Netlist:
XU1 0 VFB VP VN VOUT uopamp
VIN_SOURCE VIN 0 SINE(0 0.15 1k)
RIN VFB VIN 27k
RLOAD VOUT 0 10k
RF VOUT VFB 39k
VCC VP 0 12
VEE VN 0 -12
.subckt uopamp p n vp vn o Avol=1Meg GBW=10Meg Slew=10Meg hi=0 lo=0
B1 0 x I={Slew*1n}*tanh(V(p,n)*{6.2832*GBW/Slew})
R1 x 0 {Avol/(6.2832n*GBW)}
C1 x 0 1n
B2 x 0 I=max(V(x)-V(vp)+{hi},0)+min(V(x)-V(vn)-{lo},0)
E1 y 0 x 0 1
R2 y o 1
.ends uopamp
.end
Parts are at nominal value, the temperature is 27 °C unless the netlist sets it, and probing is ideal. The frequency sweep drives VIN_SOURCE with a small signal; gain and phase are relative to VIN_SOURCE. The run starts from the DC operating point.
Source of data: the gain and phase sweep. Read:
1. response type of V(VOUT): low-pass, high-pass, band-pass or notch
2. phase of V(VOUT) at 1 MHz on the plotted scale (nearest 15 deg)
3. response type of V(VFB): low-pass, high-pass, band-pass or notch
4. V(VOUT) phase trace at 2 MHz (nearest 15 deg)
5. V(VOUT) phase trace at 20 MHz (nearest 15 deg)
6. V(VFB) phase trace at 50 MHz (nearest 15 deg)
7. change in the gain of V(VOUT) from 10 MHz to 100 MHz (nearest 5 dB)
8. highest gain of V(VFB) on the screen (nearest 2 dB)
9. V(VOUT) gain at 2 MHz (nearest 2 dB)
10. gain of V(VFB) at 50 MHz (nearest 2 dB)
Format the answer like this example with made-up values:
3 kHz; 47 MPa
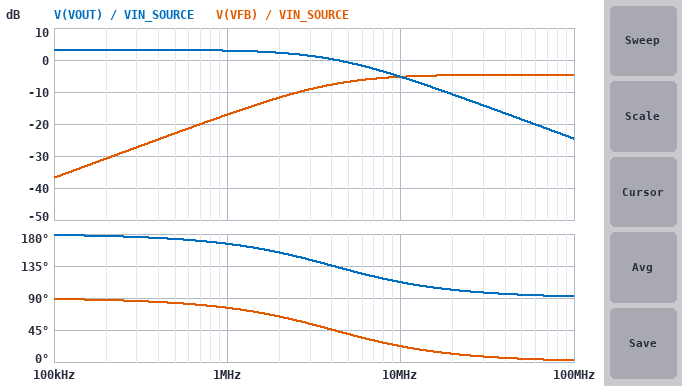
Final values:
low-pass; 165 deg; high-pass; 150 deg; 105 deg; 0 deg; -20 dB; -4 dB; 2 dB; -4 dB
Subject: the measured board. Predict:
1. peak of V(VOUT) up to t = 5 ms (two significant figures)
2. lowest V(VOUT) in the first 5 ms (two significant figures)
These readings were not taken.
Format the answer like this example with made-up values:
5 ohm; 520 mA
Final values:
220 mV; -220 mV
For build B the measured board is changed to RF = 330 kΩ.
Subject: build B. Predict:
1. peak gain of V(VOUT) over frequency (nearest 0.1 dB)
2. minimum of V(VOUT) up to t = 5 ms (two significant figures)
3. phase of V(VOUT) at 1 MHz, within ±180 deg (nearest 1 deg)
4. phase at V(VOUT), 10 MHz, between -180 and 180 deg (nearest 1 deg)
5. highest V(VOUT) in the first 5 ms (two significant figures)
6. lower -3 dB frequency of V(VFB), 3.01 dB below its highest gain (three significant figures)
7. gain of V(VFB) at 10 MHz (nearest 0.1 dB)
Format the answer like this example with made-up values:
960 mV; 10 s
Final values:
21.7 dB; -1.8 V; 127 deg; 94 deg; 1.8 V; 756 kHz; -0.7 dB
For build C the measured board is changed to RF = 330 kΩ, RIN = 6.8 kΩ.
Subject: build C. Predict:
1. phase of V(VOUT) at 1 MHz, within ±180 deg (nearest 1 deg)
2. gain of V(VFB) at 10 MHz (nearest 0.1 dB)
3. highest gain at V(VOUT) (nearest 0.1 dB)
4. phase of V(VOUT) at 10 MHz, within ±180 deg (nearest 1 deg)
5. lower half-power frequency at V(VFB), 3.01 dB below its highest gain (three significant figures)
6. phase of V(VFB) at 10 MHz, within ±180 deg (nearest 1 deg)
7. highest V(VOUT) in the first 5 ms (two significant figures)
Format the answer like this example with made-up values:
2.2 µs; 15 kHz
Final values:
101 deg; -0.2 dB; 33.7 dB; 91 deg; 202 kHz; 1 deg; 7.3 V
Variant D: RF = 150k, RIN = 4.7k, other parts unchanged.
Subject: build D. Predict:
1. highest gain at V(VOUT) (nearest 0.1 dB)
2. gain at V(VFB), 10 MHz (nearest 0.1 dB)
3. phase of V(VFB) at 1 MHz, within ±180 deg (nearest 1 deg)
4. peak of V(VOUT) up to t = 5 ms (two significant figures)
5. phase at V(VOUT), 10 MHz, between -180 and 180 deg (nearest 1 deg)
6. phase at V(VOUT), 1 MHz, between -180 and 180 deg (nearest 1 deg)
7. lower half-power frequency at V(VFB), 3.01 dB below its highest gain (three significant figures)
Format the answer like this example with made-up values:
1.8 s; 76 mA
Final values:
30.1 dB; -0.3 dB; 17 deg; 4.8 V; 92 deg; 107 deg; 304 kHz
